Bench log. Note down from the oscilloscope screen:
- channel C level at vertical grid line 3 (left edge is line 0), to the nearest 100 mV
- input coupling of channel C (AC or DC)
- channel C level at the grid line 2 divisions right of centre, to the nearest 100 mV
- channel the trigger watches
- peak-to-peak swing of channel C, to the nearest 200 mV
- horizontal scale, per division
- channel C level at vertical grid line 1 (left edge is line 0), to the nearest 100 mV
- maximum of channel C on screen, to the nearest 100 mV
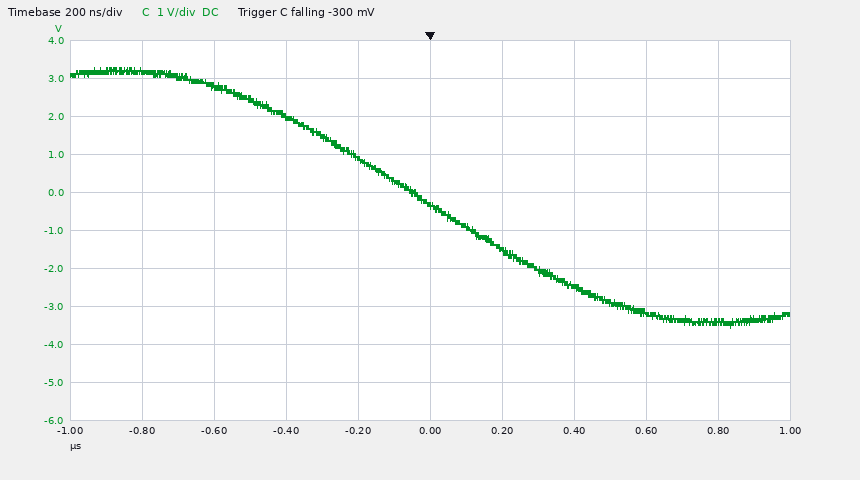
2.0 V
DC
-2.5 V
channel C
6.8 V
200 ns
3.2 V
3.3 V
